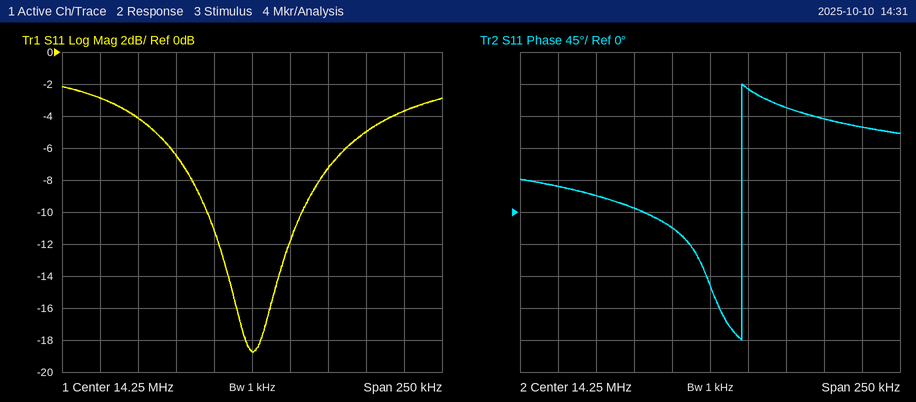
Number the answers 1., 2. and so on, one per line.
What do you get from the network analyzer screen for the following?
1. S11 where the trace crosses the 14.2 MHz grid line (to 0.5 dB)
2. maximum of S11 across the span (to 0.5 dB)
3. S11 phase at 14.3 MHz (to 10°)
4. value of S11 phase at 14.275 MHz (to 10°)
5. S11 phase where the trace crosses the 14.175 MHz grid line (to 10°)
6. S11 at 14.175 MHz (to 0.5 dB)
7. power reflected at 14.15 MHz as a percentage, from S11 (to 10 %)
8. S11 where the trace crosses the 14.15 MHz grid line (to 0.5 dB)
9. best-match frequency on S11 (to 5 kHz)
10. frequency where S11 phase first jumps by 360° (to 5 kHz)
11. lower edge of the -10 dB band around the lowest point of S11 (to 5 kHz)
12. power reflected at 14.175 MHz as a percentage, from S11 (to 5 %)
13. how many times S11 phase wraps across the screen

1. -6.5 dB
2. -2.0 dB
3. 150°
4. 170°
5. 20°
6. -4.0 dB
7. 50 %
8. -3.0 dB
9. 14.250 MHz
10. 14.270 MHz
11. 14.220 MHz
12. 40 %
13. 1
